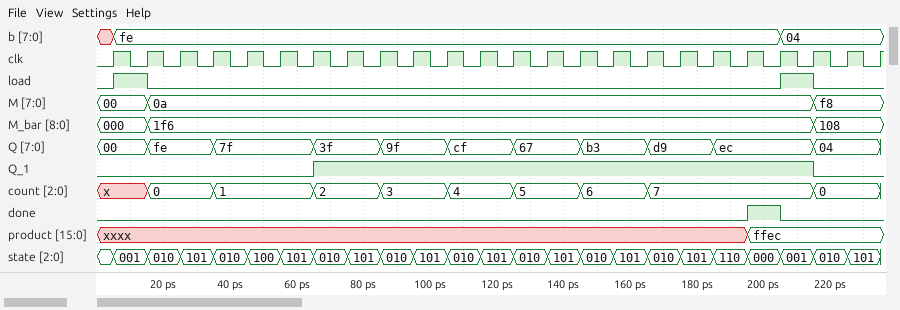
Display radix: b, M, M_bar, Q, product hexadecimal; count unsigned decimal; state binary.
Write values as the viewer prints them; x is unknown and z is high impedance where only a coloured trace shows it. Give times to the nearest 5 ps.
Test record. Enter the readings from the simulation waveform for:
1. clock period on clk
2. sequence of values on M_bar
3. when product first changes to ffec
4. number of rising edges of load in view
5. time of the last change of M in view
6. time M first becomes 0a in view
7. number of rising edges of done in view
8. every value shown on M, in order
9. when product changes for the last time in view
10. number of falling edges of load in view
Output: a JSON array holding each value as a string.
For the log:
["10 ps", "000, 1f6, 108", "195 ps", "2", "215 ps", "15 ps", "1", "00, 0a, f8", "195 ps", "2"]
